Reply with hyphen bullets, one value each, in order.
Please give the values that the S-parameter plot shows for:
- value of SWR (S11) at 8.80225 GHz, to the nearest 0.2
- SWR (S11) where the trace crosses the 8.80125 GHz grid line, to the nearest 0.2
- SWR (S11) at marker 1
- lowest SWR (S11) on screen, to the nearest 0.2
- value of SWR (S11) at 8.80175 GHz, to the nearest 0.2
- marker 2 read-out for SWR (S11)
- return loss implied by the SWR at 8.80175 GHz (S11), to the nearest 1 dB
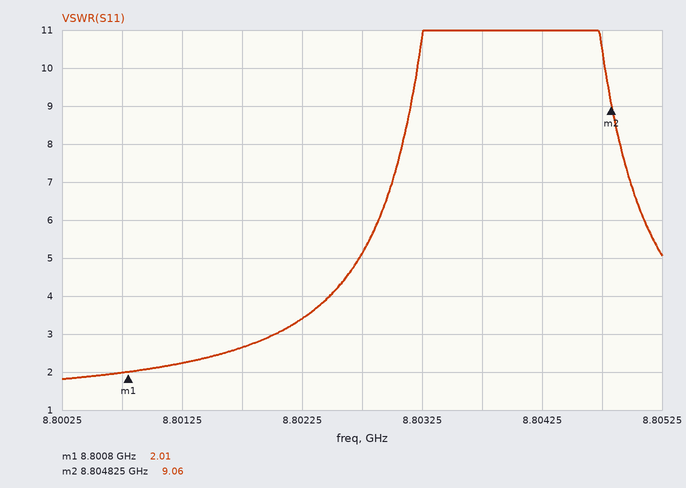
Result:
- 3.4
- 2.2
- 2.01
- 1.8
- 2.6
- 9.06
- 7 dB
